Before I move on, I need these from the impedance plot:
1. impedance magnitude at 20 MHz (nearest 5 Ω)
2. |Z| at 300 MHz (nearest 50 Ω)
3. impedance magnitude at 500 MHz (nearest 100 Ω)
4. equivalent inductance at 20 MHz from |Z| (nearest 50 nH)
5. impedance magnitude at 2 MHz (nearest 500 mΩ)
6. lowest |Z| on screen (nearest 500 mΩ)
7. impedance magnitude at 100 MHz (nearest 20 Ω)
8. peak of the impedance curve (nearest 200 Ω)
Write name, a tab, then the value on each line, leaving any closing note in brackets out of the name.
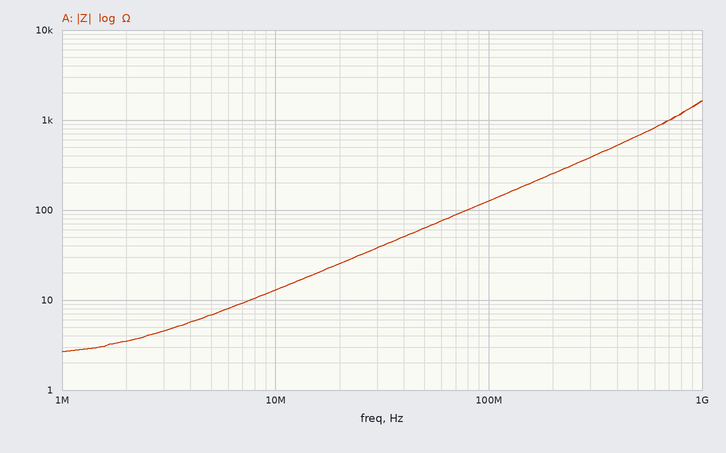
impedance magnitude at 20 MHz	25 Ω
|Z| at 300 MHz	400 Ω
impedance magnitude at 500 MHz	700 Ω
equivalent inductance at 20 MHz from |Z|	200 nH
impedance magnitude at 2 MHz	3.5 Ω
lowest |Z| on screen	2.5 Ω
impedance magnitude at 100 MHz	120 Ω
peak of the impedance curve	1.6 kΩ
